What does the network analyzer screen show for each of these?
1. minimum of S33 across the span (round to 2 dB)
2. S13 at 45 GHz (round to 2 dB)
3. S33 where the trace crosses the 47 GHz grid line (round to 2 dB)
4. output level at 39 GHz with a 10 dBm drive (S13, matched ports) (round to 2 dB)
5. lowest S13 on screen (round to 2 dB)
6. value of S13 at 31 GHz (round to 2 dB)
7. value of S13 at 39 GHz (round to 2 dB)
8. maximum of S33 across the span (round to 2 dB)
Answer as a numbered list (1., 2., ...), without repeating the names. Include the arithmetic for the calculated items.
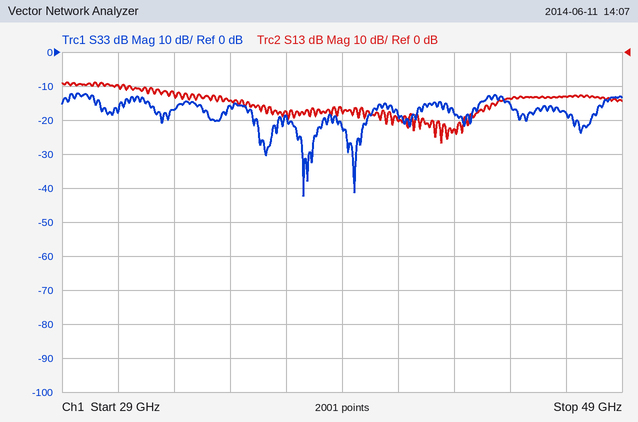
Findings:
1. -42 dB
2. -14 dB
3. -18 dB
4. 10 dBm + (-18 dB) = -8 dBm
5. -26 dB
6. -10 dB
7. -18 dB
8. -12 dB
